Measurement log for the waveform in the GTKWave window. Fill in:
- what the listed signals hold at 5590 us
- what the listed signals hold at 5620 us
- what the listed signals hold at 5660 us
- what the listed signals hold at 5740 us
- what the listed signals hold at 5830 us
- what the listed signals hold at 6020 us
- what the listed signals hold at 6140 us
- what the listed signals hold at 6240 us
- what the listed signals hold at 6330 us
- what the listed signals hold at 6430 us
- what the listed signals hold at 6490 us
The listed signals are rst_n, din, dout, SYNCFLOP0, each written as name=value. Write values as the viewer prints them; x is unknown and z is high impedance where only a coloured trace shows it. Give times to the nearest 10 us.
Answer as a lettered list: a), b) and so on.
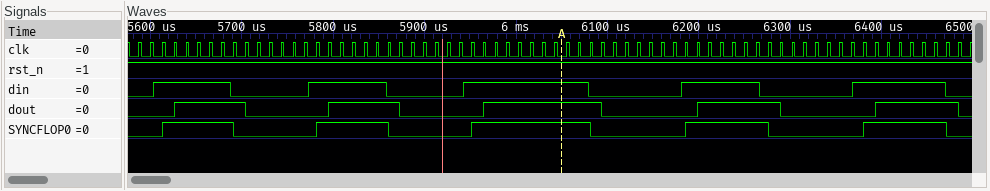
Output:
a) rst_n=1, din=0, dout=0, SYNCFLOP0=0
b) rst_n=1, din=1, dout=0, SYNCFLOP0=1
c) rst_n=1, din=1, dout=1, SYNCFLOP0=1
d) rst_n=1, din=0, dout=0, SYNCFLOP0=0
e) rst_n=1, din=1, dout=1, SYNCFLOP0=1
f) rst_n=1, din=1, dout=1, SYNCFLOP0=1
g) rst_n=1, din=0, dout=0, SYNCFLOP0=0
h) rst_n=1, din=1, dout=1, SYNCFLOP0=1
i) rst_n=1, din=0, dout=0, SYNCFLOP0=0
j) rst_n=1, din=1, dout=1, SYNCFLOP0=1
k) rst_n=1, din=0, dout=0, SYNCFLOP0=0
